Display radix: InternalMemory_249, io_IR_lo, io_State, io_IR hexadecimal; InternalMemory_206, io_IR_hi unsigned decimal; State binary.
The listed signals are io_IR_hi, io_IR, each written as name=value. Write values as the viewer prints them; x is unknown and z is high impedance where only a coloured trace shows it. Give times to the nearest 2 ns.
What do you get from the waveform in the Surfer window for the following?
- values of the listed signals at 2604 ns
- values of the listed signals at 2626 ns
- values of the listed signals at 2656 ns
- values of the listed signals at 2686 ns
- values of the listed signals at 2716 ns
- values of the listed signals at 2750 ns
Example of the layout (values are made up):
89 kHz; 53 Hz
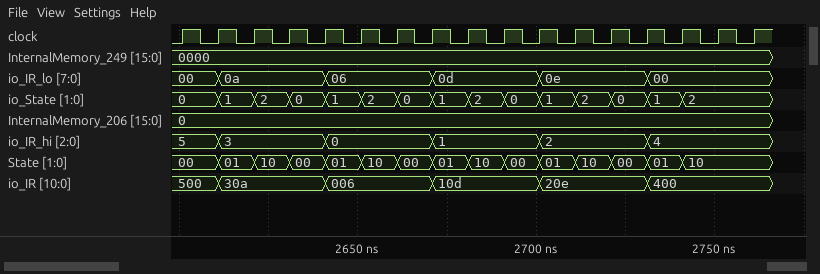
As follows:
io_IR_hi=5, io_IR=500; io_IR_hi=3, io_IR=30a; io_IR_hi=0, io_IR=006; io_IR_hi=1, io_IR=10d; io_IR_hi=2, io_IR=20e; io_IR_hi=4, io_IR=400
